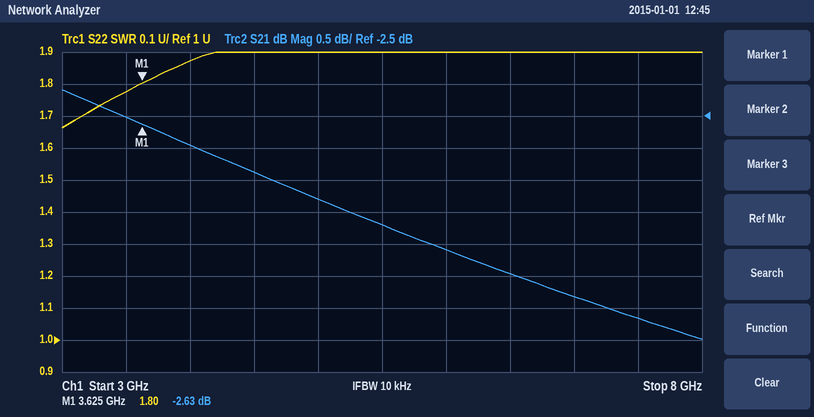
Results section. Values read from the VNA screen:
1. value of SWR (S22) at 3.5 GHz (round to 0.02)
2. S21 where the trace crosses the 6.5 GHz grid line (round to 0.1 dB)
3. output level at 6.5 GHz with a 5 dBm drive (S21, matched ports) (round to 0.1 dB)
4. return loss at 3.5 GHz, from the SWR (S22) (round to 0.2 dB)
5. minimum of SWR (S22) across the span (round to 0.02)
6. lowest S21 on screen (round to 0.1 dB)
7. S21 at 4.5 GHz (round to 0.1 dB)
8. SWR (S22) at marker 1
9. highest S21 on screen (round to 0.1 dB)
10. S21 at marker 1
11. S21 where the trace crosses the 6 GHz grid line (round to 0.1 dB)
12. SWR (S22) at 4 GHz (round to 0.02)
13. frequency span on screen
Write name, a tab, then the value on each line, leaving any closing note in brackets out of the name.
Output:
value of SWR (S22) at 3.5 GHz	1.78
S21 where the trace crosses the 6.5 GHz grid line	-5.0 dB
output level at 6.5 GHz with a 5 dBm drive (S21, matched ports)	0.0 dBm
return loss at 3.5 GHz, from the SWR (S22)	11.0 dB
minimum of SWR (S22) across the span	1.66
lowest S21 on screen	-6.0 dB
S21 at 4.5 GHz	-3.4 dB
SWR (S22) at marker 1	1.80
highest S21 on screen	-2.1 dB
S21 at marker 1	-2.63 dB
S21 where the trace crosses the 6 GHz grid line	-4.6 dB
SWR (S22) at 4 GHz	1.88
frequency span on screen	5 GHz
